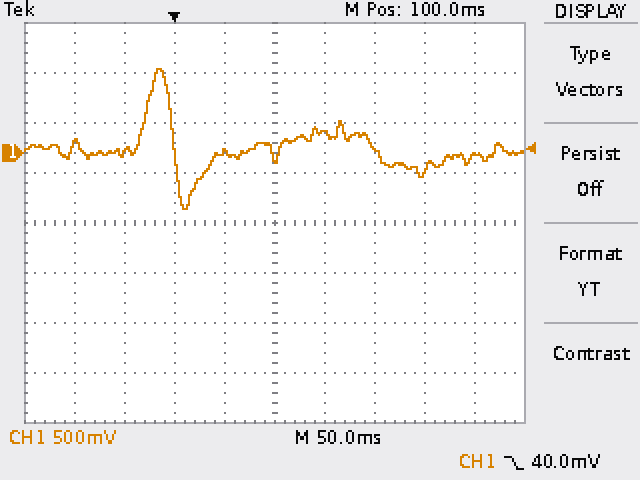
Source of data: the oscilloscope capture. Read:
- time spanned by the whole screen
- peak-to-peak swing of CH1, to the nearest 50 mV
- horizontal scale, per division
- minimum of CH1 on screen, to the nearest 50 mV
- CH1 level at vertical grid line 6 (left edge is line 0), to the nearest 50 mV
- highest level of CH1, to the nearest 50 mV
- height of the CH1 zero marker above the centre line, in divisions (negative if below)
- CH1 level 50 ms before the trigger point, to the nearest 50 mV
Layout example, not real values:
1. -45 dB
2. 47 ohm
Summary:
1. 500 ms
2. 1.40 V
3. 50 ms
4. -550 mV
5. 200 mV
6. 850 mV
7. +1.4 div
8. 0 mV
